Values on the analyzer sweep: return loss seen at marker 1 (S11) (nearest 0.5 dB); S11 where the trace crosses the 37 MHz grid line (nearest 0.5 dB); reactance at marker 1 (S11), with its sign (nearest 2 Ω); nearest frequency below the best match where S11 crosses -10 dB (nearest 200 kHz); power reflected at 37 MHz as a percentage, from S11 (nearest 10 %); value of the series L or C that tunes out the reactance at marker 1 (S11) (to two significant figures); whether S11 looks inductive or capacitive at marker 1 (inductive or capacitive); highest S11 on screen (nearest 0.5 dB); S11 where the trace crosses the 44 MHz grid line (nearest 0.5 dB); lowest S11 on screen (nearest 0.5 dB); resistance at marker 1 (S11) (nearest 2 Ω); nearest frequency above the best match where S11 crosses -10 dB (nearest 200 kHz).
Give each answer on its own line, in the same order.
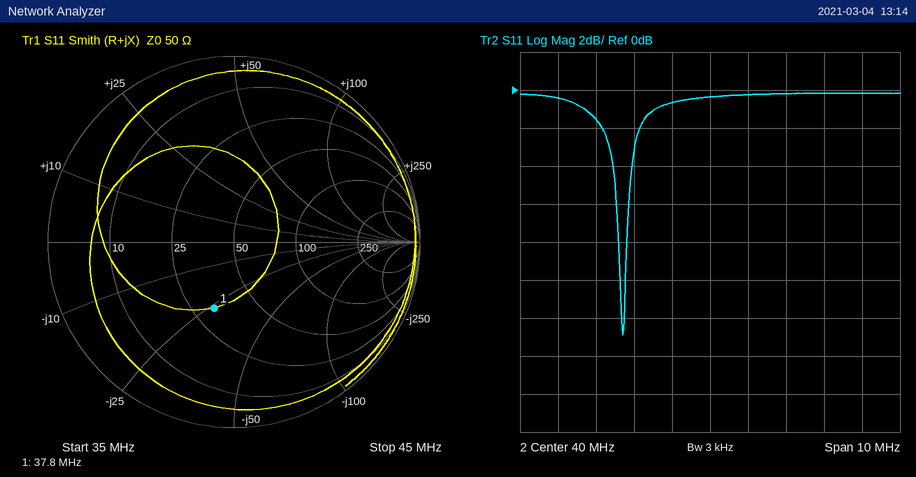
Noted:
8.5 dB
-1.5 dB
-26 Ω
37.6 MHz
70 %
110 nH
capacitive
0.0 dB
0.0 dB
-13.0 dB
32 Ω
37.8 MHz
